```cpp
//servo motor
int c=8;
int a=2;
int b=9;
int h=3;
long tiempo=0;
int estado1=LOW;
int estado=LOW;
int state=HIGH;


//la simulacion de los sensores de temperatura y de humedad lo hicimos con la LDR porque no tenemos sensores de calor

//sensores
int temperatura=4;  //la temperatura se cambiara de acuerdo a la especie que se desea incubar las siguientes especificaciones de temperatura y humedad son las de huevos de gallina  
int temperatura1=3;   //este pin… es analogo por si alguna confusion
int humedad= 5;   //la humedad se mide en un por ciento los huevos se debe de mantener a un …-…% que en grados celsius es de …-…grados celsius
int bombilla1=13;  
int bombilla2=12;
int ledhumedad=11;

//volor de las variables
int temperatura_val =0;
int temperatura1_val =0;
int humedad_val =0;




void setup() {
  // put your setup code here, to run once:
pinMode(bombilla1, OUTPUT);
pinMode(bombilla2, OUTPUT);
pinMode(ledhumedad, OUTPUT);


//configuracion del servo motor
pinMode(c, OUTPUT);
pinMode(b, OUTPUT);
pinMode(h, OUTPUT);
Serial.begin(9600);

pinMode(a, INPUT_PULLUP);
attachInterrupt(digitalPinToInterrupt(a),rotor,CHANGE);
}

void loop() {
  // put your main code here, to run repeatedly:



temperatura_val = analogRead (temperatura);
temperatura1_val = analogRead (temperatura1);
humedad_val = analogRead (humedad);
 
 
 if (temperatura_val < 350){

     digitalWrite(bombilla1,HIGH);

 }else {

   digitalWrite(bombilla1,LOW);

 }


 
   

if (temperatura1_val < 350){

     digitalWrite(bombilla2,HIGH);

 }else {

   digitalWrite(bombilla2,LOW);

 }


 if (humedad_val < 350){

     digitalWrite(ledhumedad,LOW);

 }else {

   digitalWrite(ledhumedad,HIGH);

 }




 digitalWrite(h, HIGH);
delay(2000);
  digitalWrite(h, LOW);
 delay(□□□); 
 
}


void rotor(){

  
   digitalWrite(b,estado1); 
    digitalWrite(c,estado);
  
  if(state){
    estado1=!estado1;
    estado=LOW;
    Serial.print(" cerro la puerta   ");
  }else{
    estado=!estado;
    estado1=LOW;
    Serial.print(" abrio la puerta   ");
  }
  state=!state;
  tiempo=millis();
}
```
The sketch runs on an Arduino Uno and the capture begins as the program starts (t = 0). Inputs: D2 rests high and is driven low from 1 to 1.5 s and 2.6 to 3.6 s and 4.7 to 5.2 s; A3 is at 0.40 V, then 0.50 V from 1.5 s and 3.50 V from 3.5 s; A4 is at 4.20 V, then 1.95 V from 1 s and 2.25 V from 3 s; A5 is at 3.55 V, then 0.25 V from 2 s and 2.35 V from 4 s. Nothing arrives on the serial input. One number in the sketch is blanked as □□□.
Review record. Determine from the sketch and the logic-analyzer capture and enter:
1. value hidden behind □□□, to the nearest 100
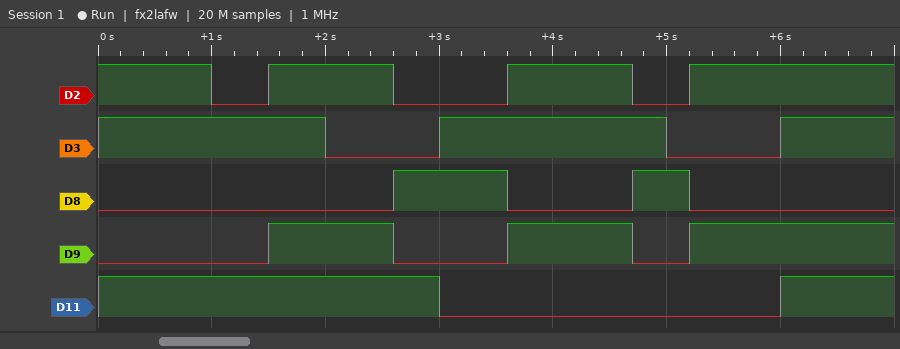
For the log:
1000
